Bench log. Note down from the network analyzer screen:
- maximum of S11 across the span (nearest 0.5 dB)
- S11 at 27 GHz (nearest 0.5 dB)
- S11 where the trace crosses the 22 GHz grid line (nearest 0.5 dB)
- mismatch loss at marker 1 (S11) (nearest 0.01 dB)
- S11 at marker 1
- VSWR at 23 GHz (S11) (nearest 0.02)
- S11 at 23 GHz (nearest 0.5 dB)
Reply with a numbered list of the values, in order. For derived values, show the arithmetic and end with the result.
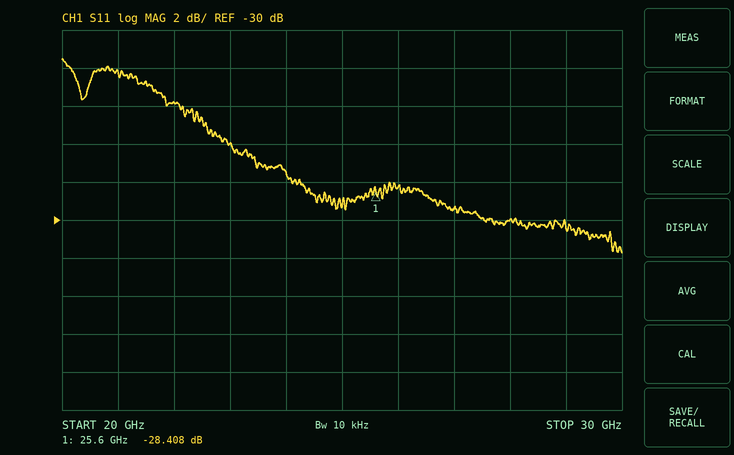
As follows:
1. -21.5 dB
2. -29.5 dB
3. -24.0 dB
4. −10 log10(1 − 10^(-28.408/10)) ≈ 0.01 dB
5. -28.408 dB
6. |Γ| = 10^(-26/20) = 0.0501; VSWR = (1 + 0.0501)/(1 − 0.0501) ≈ 1.11, so 1.10 to the nearest 0.02
7. -26.0 dB
